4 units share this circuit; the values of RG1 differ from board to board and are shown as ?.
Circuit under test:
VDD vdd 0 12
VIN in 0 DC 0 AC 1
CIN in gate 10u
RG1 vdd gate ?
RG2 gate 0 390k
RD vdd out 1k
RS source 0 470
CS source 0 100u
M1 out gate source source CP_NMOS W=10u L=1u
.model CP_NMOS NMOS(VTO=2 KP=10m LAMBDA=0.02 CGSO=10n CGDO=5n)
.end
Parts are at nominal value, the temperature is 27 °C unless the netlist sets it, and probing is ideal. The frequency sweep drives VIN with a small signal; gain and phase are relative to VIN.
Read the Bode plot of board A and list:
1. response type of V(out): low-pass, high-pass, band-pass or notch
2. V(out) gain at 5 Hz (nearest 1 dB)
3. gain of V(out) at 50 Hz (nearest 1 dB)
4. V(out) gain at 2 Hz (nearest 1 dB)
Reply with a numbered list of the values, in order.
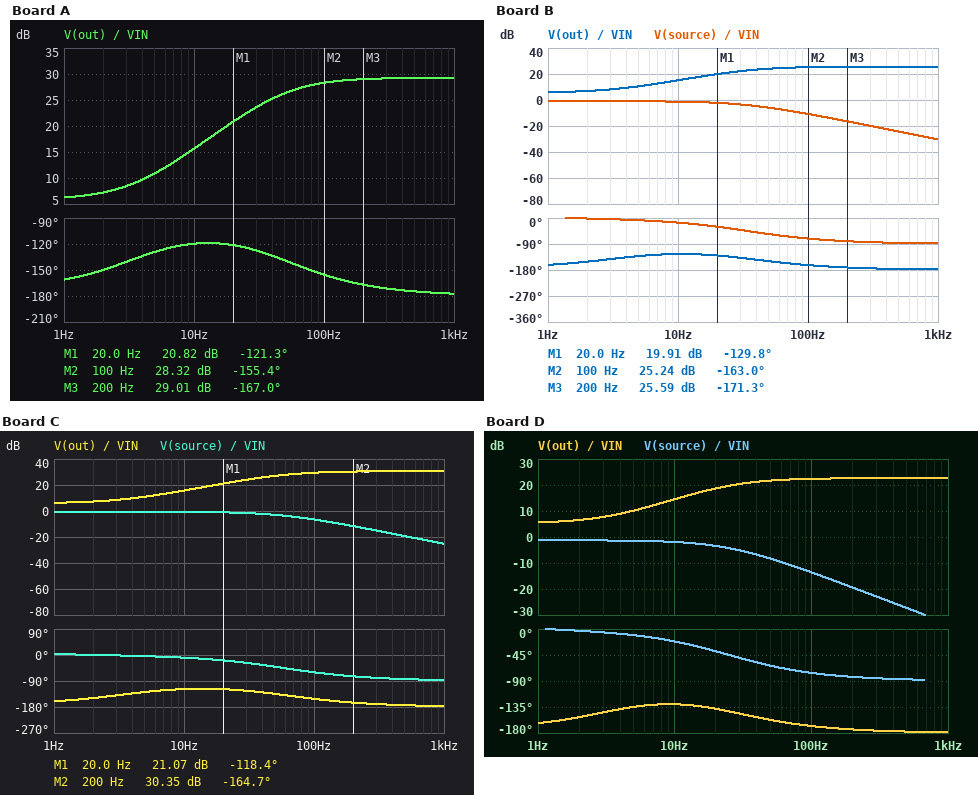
1. high-pass
2. 11 dB
3. 26 dB
4. 7 dB
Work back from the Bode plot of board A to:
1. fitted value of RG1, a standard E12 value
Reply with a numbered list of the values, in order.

1. 680 kΩ
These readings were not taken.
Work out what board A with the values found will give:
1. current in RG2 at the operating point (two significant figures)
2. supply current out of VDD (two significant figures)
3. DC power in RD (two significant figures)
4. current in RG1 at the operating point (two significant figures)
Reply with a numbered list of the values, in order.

1. 11 µA
2. 4.5 mA
3. 20 mW
4. 11 µA
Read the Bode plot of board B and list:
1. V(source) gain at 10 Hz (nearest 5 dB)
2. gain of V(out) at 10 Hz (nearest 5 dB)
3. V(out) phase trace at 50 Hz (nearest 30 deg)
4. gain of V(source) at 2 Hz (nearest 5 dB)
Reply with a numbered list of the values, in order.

1. 0 dB
2. 15 dB
3. -150 deg
4. 0 dB
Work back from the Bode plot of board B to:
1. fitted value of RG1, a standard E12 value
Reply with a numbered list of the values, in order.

1. 1.2 MΩ
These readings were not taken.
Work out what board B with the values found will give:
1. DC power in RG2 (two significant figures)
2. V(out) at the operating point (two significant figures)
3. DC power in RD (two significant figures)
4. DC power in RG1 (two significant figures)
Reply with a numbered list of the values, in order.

1. 22 µW
2. 10 V
3. 2.7 mW
4. 68 µW
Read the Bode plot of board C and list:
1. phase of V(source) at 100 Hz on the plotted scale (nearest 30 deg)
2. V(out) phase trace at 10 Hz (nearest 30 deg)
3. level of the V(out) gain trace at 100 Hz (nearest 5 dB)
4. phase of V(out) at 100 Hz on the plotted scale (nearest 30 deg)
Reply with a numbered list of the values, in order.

1. -60 deg
2. -120 deg
3. 30 dB
4. -150 deg
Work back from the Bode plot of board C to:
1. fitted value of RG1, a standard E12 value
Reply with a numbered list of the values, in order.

1. 390 kΩ
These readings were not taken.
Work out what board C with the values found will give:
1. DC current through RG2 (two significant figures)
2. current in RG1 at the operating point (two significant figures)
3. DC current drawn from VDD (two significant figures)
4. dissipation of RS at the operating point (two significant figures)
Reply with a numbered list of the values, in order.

1. 15 µA
2. 15 µA
3. 7.7 mA
4. 28 mW
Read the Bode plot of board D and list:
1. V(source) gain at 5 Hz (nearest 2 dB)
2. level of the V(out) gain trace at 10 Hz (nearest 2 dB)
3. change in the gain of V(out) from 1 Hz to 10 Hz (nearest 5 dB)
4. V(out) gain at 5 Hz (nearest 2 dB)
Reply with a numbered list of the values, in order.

1. -2 dB
2. 14 dB
3. 10 dB
4. 10 dB
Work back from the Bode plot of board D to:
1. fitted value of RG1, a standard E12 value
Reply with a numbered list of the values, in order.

1. 1.5 MΩ
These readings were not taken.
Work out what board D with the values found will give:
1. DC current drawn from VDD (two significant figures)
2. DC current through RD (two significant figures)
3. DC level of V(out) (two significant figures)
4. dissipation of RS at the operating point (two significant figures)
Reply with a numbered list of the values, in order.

1. 780 µA
2. 770 µA
3. 11 V
4. 280 µW
